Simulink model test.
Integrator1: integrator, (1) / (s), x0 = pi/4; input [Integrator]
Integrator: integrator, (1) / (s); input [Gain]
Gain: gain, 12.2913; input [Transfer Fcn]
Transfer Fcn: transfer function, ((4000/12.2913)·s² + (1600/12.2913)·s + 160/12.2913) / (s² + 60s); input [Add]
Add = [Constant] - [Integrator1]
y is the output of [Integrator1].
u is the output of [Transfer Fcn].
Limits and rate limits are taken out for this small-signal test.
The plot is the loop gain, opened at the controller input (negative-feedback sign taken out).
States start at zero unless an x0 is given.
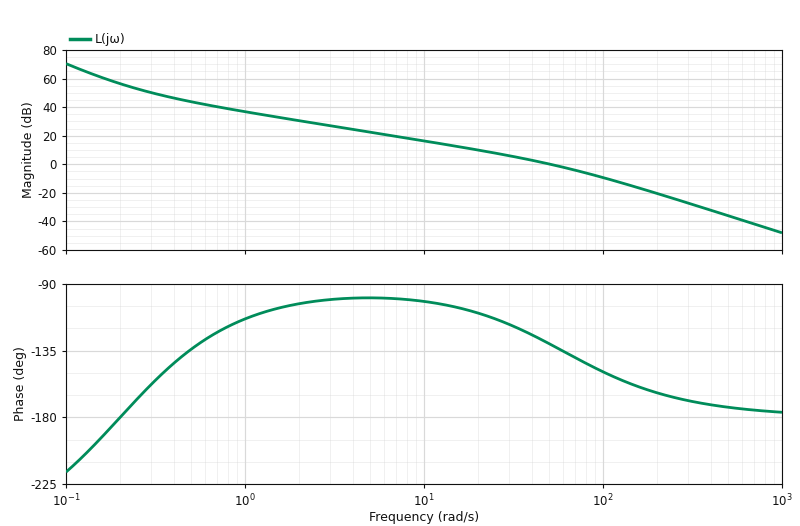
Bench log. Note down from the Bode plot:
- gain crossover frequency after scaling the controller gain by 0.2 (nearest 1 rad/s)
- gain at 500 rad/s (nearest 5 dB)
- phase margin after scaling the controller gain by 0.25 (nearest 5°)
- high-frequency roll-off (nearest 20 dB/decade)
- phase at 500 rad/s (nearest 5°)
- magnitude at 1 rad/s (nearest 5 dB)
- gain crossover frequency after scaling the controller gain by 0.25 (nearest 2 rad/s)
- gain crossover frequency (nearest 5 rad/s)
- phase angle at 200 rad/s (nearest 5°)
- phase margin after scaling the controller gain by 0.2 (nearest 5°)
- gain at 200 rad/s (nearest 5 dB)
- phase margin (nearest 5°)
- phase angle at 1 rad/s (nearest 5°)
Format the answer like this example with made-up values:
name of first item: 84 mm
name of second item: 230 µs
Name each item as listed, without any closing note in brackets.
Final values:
gain crossover frequency after scaling the controller gain by 0.2: 13 rad/s
gain at 500 rad/s: -35 dB
phase margin after scaling the controller gain by 0.25: 75°
high-frequency roll-off: -40 dB/decade
phase at 500 rad/s: -175°
magnitude at 1 rad/s: 35 dB
gain crossover frequency after scaling the controller gain by 0.25: 16 rad/s
gain crossover frequency: 50 rad/s
phase angle at 200 rad/s: -165°
phase margin after scaling the controller gain by 0.2: 75°
gain at 200 rad/s: -20 dB
phase margin: 50°
phase angle at 1 rad/s: -115°
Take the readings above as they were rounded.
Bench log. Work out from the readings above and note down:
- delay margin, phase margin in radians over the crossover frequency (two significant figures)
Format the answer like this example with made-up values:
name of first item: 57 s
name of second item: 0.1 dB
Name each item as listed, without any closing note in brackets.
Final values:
delay margin, phase margin in radians over the crossover frequency: 0.017 s
